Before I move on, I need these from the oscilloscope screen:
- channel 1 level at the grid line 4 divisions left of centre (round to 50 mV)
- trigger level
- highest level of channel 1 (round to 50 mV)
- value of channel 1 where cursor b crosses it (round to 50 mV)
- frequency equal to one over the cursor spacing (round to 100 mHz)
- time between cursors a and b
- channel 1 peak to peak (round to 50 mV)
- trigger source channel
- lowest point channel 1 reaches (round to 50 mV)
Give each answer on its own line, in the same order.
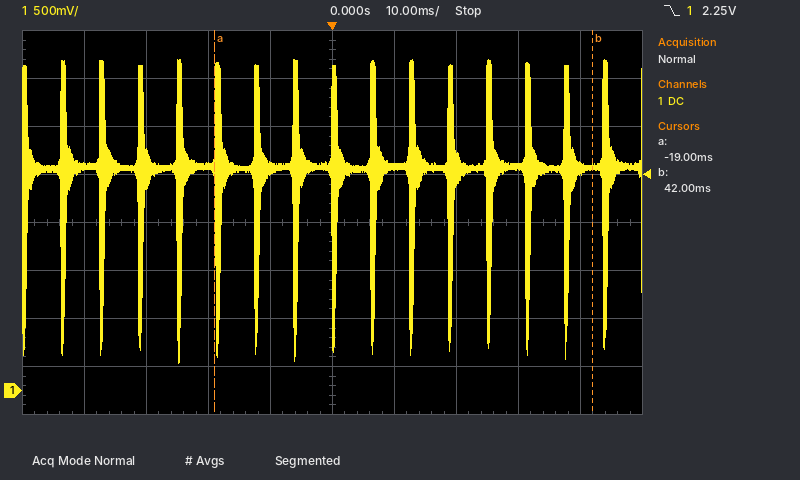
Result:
2.35 V
2.25 V
3.45 V
2.35 V
16.4 Hz
61 ms
3.15 V
channel 1
300 mV
